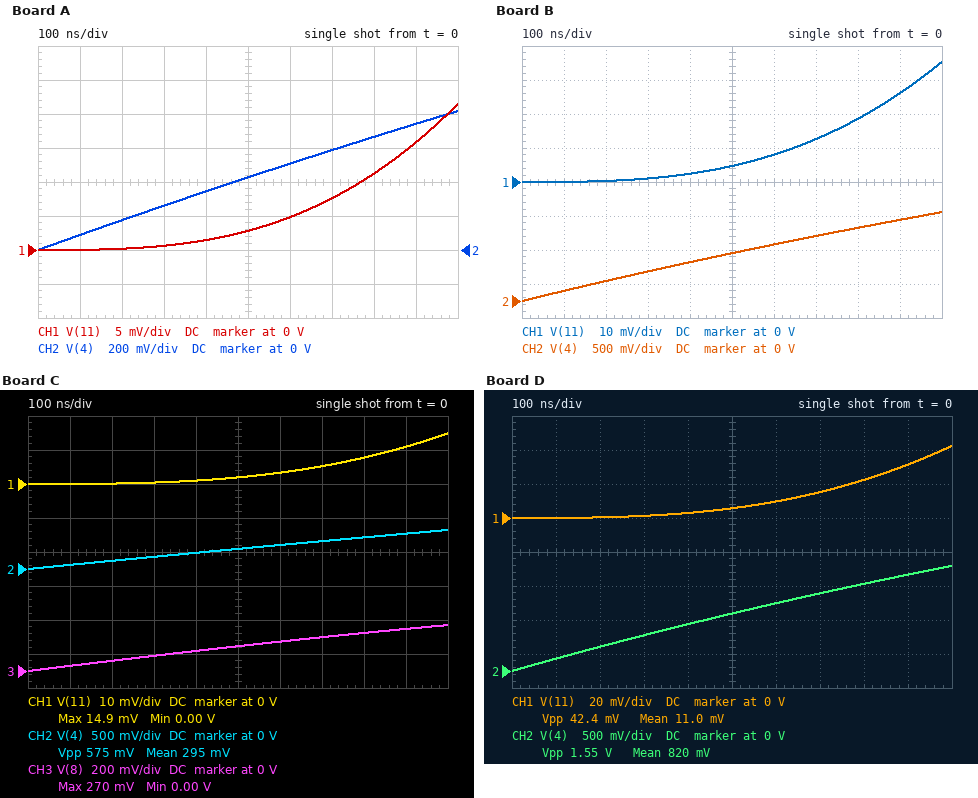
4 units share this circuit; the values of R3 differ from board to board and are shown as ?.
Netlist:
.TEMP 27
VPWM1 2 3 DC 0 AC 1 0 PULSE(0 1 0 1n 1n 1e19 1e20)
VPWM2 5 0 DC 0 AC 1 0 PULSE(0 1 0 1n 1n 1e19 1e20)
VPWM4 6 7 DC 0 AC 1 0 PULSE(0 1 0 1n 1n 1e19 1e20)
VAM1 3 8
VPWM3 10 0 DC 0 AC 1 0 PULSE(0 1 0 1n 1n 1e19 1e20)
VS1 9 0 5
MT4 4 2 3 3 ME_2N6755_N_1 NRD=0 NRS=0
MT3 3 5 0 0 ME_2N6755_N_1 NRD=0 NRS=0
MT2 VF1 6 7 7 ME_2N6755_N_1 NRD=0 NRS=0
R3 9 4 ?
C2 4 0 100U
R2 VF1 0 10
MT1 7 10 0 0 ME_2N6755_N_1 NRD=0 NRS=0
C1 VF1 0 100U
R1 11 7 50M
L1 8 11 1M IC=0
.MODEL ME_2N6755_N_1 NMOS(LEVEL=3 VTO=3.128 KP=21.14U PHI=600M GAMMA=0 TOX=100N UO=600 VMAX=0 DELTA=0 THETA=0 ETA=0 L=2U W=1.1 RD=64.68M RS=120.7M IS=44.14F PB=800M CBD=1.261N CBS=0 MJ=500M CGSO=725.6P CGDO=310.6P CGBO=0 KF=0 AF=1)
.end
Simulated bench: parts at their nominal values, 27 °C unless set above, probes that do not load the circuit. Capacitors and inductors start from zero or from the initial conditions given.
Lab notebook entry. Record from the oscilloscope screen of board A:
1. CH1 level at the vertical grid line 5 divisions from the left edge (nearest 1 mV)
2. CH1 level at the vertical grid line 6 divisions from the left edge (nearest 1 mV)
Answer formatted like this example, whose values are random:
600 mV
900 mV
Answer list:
3 mV
5 mV
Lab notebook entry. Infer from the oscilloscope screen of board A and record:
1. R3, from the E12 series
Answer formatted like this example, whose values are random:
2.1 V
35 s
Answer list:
0.056 Ω
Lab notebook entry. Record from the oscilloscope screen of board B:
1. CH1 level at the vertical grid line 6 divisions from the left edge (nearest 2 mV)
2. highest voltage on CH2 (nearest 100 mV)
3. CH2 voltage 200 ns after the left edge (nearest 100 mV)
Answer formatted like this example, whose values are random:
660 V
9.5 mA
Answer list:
8 mV
1.3 V
300 mV
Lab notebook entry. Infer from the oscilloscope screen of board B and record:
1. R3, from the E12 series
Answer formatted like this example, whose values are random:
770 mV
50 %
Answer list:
0.033 Ω
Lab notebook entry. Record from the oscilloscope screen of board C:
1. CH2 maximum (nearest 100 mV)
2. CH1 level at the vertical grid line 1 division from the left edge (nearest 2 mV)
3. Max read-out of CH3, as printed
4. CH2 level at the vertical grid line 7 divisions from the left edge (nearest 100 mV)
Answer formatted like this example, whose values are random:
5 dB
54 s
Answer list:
600 mV
0 V
270 mV
400 mV
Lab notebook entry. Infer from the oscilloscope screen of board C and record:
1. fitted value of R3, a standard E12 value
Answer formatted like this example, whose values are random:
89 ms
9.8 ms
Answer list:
0.082 Ω
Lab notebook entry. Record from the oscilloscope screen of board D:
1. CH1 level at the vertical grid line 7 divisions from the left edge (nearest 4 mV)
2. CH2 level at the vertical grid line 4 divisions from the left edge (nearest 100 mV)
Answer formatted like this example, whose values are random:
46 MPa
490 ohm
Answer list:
16 mV
700 mV
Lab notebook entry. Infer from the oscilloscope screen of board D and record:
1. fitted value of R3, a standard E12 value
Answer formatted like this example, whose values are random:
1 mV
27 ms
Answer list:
0.027 Ω
